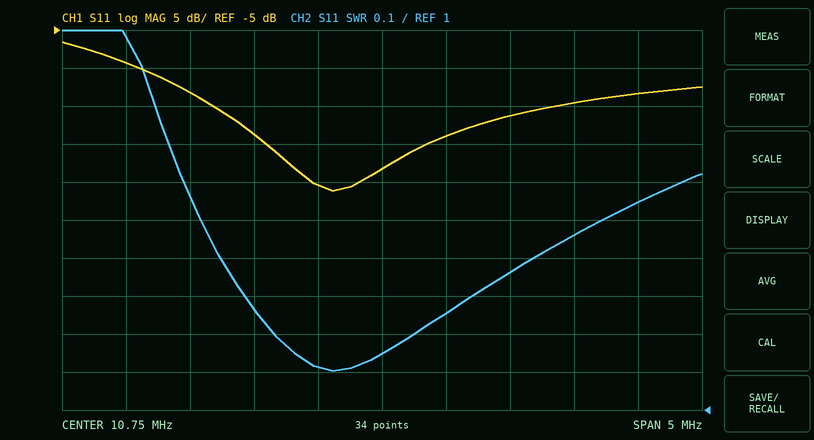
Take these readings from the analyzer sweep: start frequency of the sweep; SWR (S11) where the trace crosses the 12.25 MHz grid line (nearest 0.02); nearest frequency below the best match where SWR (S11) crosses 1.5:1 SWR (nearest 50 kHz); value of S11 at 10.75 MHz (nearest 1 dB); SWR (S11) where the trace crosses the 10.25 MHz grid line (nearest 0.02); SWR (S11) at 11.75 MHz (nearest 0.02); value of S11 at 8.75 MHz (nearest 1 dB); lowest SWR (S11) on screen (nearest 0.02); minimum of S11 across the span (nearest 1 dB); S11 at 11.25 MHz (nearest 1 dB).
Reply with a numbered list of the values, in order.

1. 8.25 MHz
2. 1.46
3. 9.35 MHz
4. -23 dB
5. 1.12
6. 1.36
7. -9 dB
8. 1.10
9. -26 dB
10. -19 dB
